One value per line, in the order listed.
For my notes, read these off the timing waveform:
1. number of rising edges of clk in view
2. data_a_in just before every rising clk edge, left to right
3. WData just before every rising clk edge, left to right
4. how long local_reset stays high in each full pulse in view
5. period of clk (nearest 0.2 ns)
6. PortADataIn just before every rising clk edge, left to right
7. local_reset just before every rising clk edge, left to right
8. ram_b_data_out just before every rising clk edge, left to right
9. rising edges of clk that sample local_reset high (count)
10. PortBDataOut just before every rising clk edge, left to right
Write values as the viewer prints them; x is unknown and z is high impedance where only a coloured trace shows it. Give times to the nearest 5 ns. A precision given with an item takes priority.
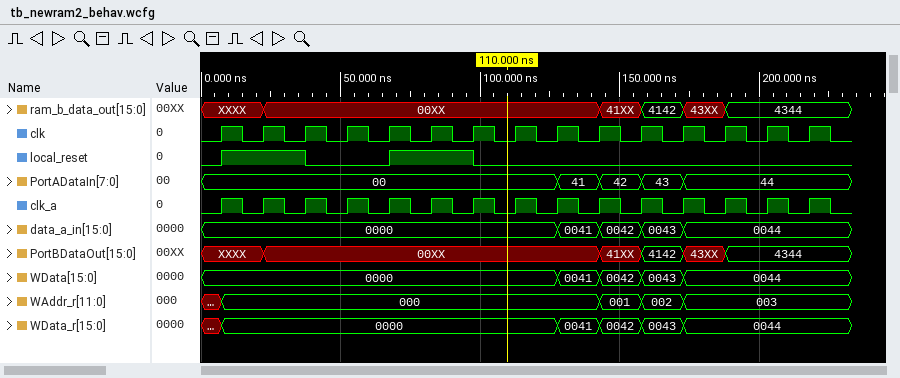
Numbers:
15
0000, 0000, 0000, 0000, 0000, 0000, 0000, 0000, 0000, 0041, 0042, 0043, 0044, 0044, 0044
0000, 0000, 0000, 0000, 0000, 0000, 0000, 0000, 0000, 0041, 0042, 0043, 0044, 0044, 0044
30 ns, 30 ns
15 ns
00, 00, 00, 00, 00, 00, 00, 00, 00, 41, 42, 43, 44, 44, 44
0 1 1 0 0 1 1 0 0 0 0 0 0 0 0
XXXX, XXXX, 00XX, 00XX, 00XX, 00XX, 00XX, 00XX, 00XX, 00XX, 41XX, 4142, 43XX, 4344, 4344
4
XXXX, XXXX, 00XX, 00XX, 00XX, 00XX, 00XX, 00XX, 00XX, 00XX, 41XX, 4142, 43XX, 4344, 4344
